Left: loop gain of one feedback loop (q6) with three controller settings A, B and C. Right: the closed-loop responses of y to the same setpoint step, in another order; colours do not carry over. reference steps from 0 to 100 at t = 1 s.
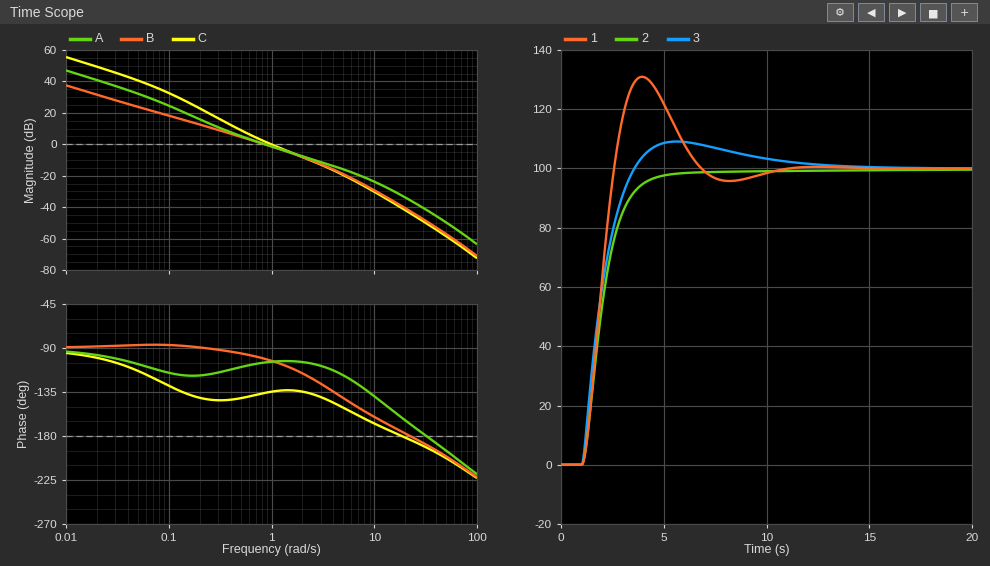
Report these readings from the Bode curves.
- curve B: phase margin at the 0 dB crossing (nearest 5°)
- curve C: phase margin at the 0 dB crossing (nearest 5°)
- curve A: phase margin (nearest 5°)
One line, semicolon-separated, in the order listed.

80°; 45°; 75°
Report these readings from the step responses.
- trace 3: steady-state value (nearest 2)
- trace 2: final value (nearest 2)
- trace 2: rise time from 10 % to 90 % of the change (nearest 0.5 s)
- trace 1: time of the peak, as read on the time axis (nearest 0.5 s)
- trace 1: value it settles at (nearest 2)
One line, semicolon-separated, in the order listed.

100; 100; 2.0 s; 4.0 s; 100
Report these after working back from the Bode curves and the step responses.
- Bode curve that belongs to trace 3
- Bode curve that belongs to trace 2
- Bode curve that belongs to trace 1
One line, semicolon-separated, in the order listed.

A; B; C
